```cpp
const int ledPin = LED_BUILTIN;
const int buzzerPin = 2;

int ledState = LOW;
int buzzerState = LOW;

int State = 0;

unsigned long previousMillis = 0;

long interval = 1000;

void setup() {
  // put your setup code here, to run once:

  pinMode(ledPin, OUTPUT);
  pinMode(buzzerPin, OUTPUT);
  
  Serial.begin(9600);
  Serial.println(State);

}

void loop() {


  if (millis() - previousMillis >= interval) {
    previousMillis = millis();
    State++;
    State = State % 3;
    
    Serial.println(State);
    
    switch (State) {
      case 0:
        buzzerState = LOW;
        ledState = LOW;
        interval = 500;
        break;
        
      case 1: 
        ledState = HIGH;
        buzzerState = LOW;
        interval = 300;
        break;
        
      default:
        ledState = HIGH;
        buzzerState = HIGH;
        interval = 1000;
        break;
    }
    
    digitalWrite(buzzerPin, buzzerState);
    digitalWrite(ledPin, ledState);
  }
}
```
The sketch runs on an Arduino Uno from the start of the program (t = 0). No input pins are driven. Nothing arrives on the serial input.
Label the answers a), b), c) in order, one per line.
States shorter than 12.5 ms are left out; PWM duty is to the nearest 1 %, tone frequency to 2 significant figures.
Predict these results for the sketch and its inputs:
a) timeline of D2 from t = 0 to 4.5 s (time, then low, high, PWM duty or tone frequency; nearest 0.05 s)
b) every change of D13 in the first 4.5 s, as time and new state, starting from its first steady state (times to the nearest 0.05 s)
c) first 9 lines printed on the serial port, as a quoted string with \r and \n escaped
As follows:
a) 0 s low; 1.3 s high; 2.3 s low; 3.1 s high; 4.1 s low
b) 0 s low; 1 s high; 2.3 s low; 2.8 s high; 4.1 s low
c) "0\r\n1\r\n2\r\n0\r\n1\r\n2\r\n0\r\n1\r\n2\r\n"
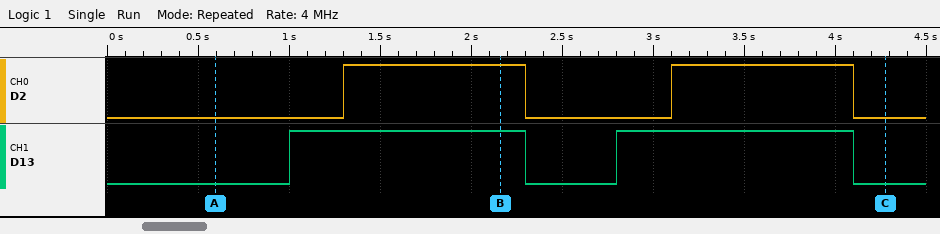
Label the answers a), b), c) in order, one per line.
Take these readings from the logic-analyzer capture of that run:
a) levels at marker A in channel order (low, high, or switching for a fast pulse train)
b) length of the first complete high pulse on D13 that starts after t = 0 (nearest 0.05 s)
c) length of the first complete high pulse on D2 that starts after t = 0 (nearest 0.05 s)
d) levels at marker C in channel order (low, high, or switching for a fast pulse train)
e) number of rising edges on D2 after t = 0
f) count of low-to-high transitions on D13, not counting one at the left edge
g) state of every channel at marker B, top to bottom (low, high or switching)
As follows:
a) D2 low, D13 low
b) 1.30 s
c) 1.00 s
d) D2 low, D13 low
e) 2
f) 2
g) D2 high, D13 high
